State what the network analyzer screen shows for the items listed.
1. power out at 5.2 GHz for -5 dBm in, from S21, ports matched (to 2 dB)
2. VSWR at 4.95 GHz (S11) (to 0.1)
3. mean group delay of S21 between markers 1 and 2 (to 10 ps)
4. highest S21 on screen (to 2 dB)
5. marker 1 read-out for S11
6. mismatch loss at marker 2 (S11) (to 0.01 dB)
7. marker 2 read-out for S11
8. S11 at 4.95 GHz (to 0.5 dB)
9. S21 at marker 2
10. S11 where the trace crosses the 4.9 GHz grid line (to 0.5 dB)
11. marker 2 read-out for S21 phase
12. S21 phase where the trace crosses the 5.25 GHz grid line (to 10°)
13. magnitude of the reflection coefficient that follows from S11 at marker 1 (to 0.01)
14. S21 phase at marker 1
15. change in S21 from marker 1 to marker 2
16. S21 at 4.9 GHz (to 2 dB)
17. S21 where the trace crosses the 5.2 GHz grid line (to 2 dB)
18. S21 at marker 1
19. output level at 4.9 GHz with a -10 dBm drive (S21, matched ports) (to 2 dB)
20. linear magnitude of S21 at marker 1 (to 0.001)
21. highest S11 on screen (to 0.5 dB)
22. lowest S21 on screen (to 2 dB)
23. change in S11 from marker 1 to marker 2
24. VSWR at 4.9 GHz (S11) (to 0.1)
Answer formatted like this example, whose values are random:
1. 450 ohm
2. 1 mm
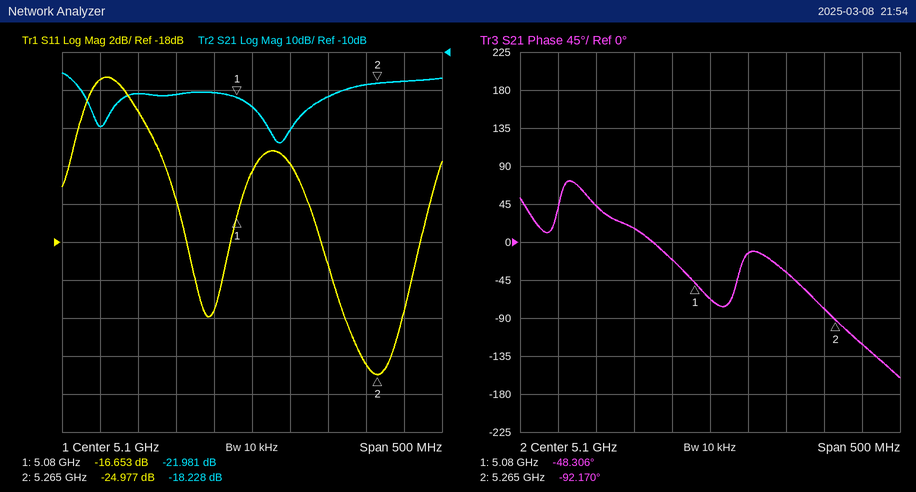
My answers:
1. -26 dBm
2. 1.8
3. 660 ps
4. -16 dB
5. -16.653 dB
6. 0.01 dB
7. -24.977 dB
8. -11.0 dB
9. -18.228 dB
10. -9.5 dB
11. -92.170°
12. -80°
13. 0.15
14. -48.306°
15. 3.753 dB
16. -30 dB
17. -22 dB
18. -21.981 dB
19. -40 dBm
20. 0.080
21. -9.5 dB
22. -34 dB
23. -8.324 dB
24. 2.0
